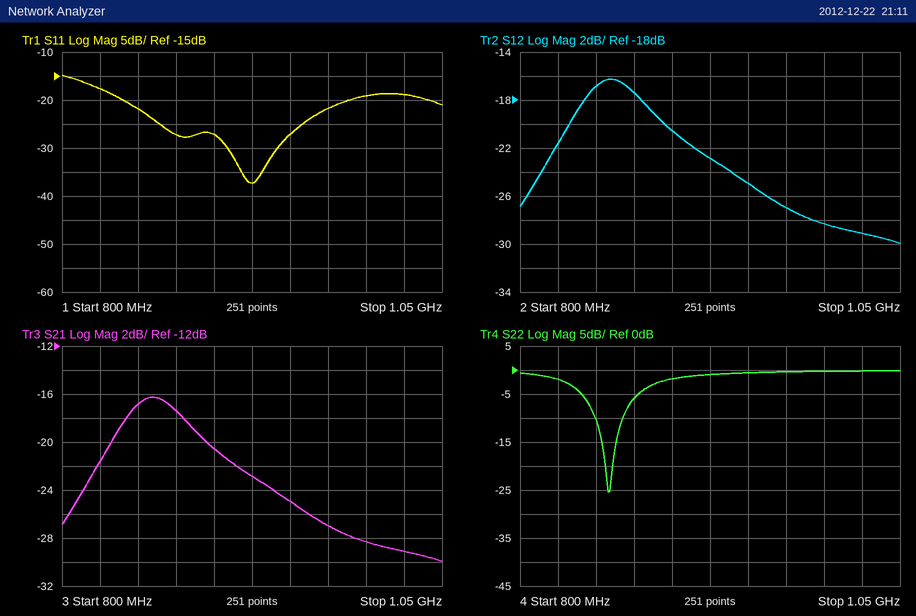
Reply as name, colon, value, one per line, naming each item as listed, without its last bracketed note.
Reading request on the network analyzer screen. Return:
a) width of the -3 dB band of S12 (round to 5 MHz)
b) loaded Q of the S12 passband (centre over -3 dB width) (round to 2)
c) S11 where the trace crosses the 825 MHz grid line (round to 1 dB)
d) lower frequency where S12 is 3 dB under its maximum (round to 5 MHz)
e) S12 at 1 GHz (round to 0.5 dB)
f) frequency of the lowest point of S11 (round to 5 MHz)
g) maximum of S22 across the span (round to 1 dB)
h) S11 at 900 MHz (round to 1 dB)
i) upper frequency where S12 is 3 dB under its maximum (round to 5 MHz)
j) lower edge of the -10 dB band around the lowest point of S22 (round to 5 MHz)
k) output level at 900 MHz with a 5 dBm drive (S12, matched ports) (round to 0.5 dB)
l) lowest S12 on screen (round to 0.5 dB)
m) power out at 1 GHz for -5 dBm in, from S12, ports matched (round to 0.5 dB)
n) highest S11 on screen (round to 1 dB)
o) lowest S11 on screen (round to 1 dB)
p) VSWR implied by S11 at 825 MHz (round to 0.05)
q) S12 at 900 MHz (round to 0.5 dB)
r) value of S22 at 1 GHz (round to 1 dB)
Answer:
width of the -3 dB band of S12: 55 MHz
loaded Q of the S12 passband (centre over -3 dB width): 16
S11 where the trace crosses the 825 MHz grid line: -18 dB
lower frequency where S12 is 3 dB under its maximum: 835 MHz
S12 at 1 GHz: -28.5 dB
frequency of the lowest point of S11: 925 MHz
maximum of S22 across the span: 0 dB
S11 at 900 MHz: -27 dB
upper frequency where S12 is 3 dB under its maximum: 890 MHz
lower edge of the -10 dB band around the lowest point of S22: 850 MHz
output level at 900 MHz with a 5 dBm drive (S12, matched ports): -15.5 dBm
lowest S12 on screen: -30.0 dB
power out at 1 GHz for -5 dBm in, from S12, ports matched: -33.5 dBm
highest S11 on screen: -15 dB
lowest S11 on screen: -37 dB
VSWR implied by S11 at 825 MHz: 1.30
S12 at 900 MHz: -20.5 dB
value of S22 at 1 GHz: 0 dB
